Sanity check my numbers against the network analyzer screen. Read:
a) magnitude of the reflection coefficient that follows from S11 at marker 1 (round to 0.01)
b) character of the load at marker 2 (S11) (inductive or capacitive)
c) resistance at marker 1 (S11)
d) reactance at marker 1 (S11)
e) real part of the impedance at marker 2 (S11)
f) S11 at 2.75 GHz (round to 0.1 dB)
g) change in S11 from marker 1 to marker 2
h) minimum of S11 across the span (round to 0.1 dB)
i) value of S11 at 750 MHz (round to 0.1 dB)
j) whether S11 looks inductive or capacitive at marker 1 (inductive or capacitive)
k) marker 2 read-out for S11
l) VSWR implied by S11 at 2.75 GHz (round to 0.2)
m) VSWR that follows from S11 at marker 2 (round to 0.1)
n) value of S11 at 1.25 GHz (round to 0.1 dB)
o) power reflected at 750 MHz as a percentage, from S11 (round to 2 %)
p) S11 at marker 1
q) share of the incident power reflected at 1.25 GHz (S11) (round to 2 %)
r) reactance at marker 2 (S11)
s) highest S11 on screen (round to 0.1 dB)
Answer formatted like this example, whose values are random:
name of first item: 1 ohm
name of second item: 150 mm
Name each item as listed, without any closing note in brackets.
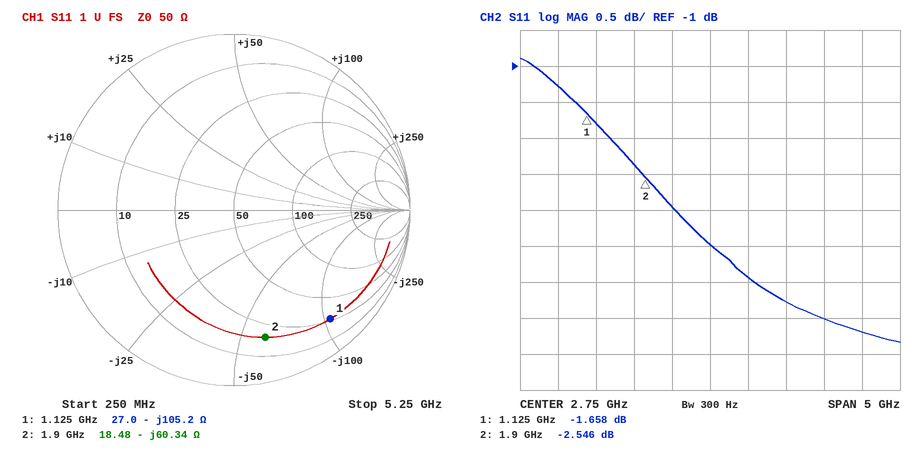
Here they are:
magnitude of the reflection coefficient that follows from S11 at marker 1: 0.83
character of the load at marker 2 (S11): capacitive
resistance at marker 1: 27.0 Ω
reactance at marker 1: -105.2 Ω
real part of the impedance at marker 2: 18.48 Ω
S11 at 2.75 GHz: -3.5 dB
change in S11 from marker 1 to marker 2: -0.888 dB
minimum of S11 across the span: -4.8 dB
value of S11 at 750 MHz: -1.3 dB
whether S11 looks inductive or capacitive at marker 1: capacitive
marker 2 read-out for S11: -2.546 dB
VSWR implied by S11 at 2.75 GHz: 5.0
VSWR that follows from S11 at marker 2: 6.9
value of S11 at 1.25 GHz: -1.8 dB
power reflected at 750 MHz as a percentage, from S11: 74 %
S11 at marker 1: -1.658 dB
share of the incident power reflected at 1.25 GHz (S11): 66 %
reactance at marker 2: -60.34 Ω
highest S11 on screen: -0.9 dB
